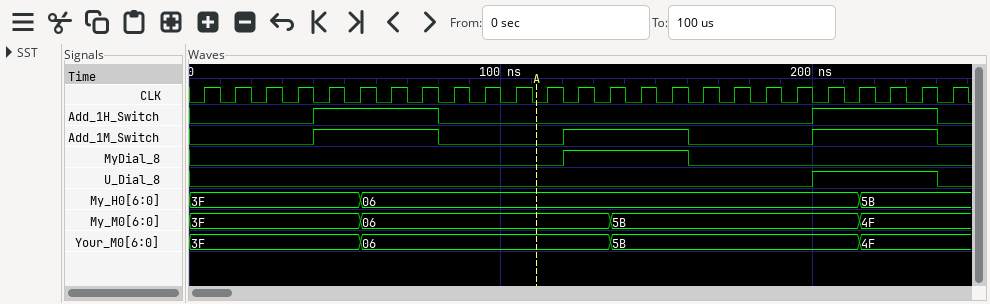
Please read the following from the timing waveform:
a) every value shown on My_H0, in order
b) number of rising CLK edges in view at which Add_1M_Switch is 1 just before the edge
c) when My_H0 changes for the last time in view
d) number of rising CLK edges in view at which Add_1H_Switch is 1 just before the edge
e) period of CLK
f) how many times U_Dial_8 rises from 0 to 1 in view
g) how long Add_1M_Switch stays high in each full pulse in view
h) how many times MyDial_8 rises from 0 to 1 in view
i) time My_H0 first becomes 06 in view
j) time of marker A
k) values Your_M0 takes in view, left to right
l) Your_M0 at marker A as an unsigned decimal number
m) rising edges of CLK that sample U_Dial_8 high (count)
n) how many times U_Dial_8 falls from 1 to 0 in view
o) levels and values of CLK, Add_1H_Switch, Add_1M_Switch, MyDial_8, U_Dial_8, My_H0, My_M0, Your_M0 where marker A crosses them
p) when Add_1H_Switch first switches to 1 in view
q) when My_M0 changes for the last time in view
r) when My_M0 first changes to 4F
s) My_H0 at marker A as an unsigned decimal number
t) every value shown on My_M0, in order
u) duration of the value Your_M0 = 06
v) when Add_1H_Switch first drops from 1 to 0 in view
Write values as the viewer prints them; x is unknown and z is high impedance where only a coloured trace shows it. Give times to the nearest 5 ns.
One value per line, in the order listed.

3F, 06, 5B
12
215 ns
8
10 ns
1
40 ns, 40 ns, 40 ns
1
55 ns
110 ns
3F, 06, 5B, 4F
6
4
1
CLK=0, Add_1H_Switch=0, Add_1M_Switch=0, MyDial_8=0, U_Dial_8=0, My_H0=06, My_M0=06, Your_M0=06
40 ns
215 ns
215 ns
6
3F, 06, 5B, 4F
80 ns
80 ns
